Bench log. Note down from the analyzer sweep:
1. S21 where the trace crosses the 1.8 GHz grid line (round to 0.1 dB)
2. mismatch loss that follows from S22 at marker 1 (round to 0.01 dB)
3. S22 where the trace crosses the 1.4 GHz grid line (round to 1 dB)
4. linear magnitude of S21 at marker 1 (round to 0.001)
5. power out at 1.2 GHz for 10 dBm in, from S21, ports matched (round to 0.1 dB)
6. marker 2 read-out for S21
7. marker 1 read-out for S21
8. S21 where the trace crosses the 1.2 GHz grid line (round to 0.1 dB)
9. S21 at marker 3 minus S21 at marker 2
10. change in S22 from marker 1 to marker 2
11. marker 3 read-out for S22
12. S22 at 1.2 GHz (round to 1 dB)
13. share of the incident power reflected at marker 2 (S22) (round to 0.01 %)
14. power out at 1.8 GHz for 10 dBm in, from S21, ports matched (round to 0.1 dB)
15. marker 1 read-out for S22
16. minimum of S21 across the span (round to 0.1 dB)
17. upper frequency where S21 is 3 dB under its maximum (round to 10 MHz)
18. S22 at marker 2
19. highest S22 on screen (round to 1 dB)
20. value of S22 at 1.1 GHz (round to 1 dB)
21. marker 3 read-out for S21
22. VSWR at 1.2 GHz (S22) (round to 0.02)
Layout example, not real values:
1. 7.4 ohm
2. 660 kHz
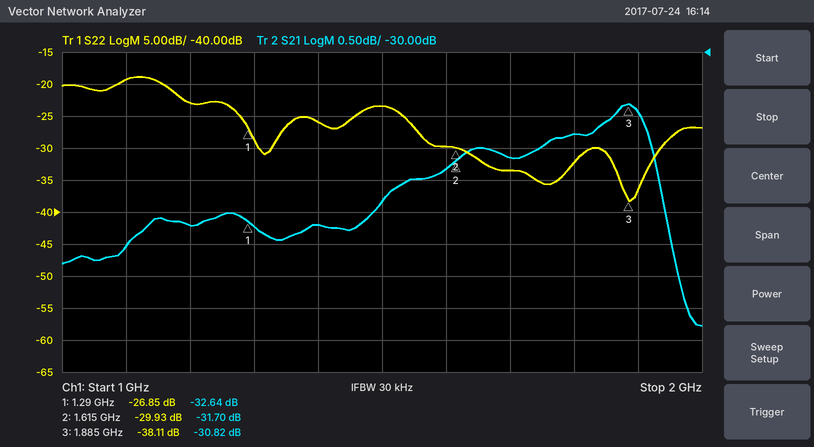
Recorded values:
1. -31.3 dB
2. 0.01 dB
3. -26 dB
4. 0.023
5. -22.7 dBm
6. -31.70 dB
7. -32.64 dB
8. -32.7 dB
9. 0.88 dB
10. -3.08 dB
11. -38.11 dB
12. -23 dB
13. 0.10 %
14. -21.3 dBm
15. -26.85 dB
16. -34.3 dB
17. 1.97 GHz
18. -29.93 dB
19. -19 dB
20. -19 dB
21. -30.82 dB
22. 1.16
